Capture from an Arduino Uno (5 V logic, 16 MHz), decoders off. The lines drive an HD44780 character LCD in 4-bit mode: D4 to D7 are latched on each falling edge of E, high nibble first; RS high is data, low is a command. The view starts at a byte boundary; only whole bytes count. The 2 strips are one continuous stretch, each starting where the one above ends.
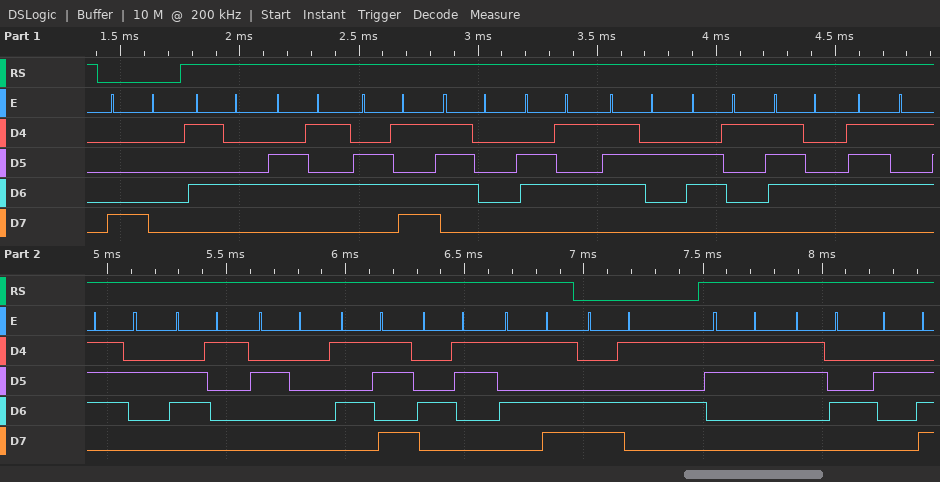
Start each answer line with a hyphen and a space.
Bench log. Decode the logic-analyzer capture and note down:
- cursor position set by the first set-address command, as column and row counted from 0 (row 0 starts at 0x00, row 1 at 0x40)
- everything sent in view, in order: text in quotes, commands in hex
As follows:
- column 0, row 0
- 0x80 "Temperatura [C]" 0xC5 "34."
